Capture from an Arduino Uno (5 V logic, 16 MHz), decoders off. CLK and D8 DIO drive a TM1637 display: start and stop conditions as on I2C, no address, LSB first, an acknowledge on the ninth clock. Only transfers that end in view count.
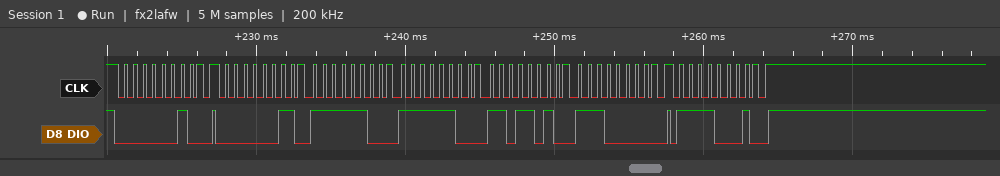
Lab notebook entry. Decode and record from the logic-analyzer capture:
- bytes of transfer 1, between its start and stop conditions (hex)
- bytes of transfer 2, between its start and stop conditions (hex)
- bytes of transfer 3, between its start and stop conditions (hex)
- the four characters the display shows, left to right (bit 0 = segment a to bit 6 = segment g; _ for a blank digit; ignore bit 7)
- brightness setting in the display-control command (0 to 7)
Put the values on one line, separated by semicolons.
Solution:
40; C0 3F 3F 5B 07; 8F; 0027; 7
